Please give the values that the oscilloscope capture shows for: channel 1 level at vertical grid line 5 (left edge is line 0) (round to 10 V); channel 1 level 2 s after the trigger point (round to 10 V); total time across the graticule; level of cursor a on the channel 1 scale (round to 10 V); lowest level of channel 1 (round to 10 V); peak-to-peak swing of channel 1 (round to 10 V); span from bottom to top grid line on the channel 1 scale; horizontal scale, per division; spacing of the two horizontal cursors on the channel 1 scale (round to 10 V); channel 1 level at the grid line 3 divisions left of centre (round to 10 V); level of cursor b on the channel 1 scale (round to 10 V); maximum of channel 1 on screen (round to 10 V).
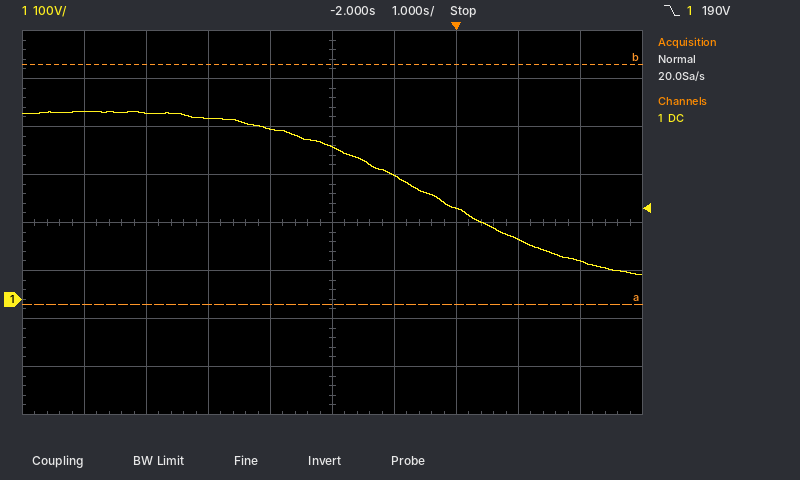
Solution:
320 V
80 V
10 s
-10 V
50 V
340 V
800 V
1 s
500 V
390 V
490 V
390 V
